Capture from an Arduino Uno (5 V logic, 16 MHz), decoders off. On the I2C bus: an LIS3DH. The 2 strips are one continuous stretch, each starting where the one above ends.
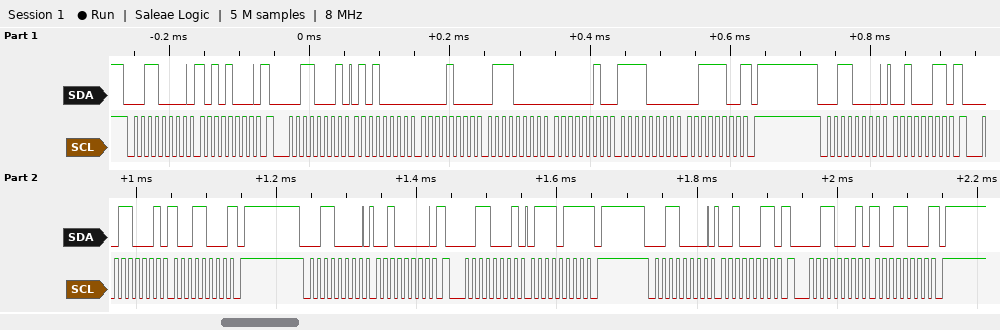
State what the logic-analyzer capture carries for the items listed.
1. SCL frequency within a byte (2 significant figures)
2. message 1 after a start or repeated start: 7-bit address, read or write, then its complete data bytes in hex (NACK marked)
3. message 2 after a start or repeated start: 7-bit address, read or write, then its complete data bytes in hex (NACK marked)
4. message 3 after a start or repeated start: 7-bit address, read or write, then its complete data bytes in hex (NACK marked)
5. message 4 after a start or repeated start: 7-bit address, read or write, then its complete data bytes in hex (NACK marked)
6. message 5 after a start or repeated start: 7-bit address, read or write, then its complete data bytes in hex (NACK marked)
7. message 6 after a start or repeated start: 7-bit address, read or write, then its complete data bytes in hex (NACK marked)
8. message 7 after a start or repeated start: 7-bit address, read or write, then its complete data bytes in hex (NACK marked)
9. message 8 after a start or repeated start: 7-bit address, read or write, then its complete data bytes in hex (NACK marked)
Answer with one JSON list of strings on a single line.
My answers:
["100 kHz", "0x18 write: A8", "0x18 read: 50 08 70 02 F0 3C NACK", "0x18 write: 23", "0x18 read: 98 NACK", "0x18 write: 20", "0x18 read: 77 NACK", "0x18 write: 23", "0x18 read: 98 NACK"]
